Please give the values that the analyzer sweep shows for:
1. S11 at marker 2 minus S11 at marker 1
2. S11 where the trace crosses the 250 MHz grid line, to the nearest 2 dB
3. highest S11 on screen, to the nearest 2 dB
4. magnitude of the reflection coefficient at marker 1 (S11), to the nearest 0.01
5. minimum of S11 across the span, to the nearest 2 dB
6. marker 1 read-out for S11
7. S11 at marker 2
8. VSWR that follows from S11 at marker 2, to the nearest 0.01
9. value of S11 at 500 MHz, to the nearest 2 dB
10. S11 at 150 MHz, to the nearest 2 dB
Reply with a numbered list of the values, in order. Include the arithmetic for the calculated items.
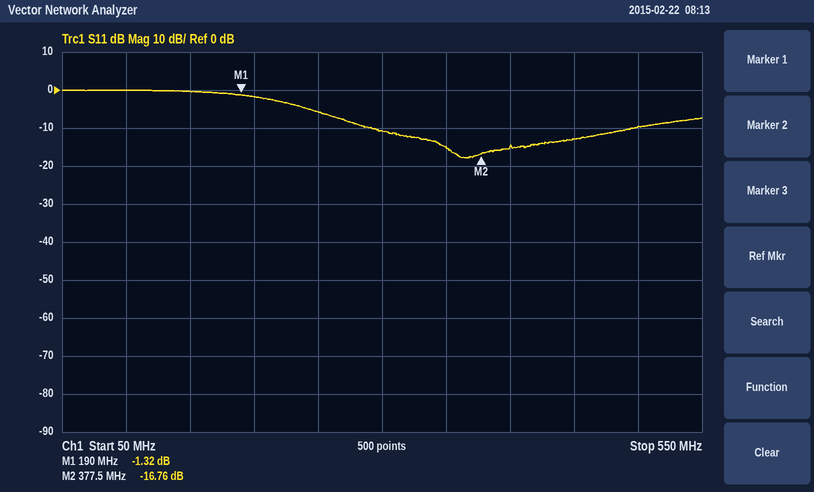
1. -16.76 − (-1.32) = -15.44 dB
2. -6 dB
3. 0 dB
4. 10^(-1.32/20) ≈ 0.86
5. -18 dB
6. -1.32 dB
7. -16.76 dB
8. (1 + 0.1452)/(1 − 0.1452) ≈ 1.34
9. -10 dB
10. 0 dB
